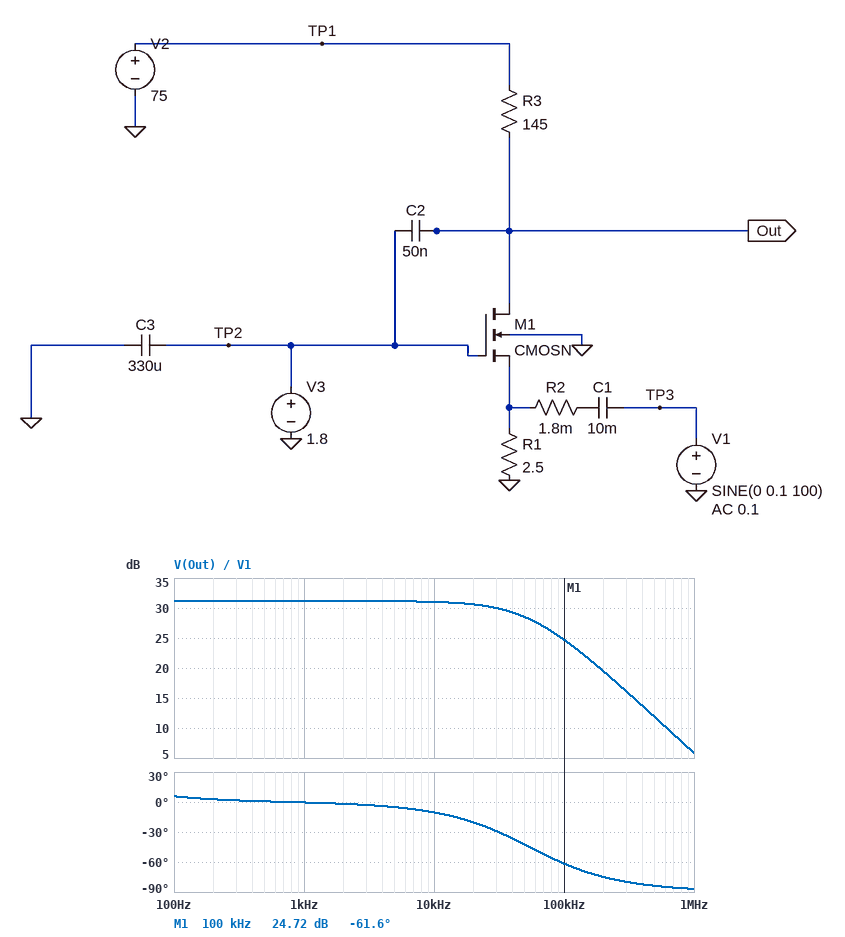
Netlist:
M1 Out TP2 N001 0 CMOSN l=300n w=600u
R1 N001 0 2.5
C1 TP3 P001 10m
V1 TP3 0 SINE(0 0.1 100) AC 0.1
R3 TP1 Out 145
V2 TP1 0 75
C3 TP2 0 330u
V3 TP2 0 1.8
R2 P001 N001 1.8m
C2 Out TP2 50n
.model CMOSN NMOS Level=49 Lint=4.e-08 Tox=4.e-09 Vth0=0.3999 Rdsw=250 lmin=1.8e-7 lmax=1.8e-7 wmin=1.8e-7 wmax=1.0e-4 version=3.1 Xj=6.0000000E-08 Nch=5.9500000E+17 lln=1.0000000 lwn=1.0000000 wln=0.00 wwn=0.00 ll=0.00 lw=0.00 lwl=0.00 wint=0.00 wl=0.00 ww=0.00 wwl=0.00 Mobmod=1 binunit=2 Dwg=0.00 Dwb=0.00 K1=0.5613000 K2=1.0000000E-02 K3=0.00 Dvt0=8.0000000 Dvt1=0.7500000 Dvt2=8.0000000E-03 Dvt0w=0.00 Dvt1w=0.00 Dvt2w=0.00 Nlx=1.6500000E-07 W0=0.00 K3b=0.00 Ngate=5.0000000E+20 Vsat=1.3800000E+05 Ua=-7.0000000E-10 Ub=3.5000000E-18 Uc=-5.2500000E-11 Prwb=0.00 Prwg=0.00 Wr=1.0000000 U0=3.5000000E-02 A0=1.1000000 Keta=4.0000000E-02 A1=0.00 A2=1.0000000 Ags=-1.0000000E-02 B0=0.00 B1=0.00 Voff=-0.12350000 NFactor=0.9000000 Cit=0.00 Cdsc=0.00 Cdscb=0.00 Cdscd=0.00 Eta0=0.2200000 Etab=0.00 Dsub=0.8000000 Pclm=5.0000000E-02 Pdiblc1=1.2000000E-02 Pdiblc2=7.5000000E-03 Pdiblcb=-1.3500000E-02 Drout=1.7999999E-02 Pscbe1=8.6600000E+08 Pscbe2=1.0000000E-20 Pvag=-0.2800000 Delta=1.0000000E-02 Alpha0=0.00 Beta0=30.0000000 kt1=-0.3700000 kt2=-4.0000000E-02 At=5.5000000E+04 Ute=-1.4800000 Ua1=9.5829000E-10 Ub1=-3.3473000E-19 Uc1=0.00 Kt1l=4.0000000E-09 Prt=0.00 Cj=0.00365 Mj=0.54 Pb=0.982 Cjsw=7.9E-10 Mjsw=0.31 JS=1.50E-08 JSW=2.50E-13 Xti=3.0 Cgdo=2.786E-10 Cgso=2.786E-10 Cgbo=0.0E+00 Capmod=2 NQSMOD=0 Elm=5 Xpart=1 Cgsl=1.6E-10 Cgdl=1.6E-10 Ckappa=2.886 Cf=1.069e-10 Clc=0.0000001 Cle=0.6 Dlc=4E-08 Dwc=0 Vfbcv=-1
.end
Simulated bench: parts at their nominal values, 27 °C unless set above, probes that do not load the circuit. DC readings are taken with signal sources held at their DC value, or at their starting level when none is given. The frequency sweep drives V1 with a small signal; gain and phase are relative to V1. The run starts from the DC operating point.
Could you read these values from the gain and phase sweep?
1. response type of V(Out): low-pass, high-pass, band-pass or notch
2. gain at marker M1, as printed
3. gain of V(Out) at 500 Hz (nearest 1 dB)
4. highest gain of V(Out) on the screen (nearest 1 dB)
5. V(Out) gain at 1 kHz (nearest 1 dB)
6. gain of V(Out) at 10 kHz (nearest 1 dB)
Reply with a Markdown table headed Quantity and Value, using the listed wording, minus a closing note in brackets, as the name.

| Quantity | Value |
|---|---|
| response type of V(Out): low-pass, high-pass, band-pass or notch | low-pass |
| gain at marker M1, as printed | 24.72 dB |
| gain of V(Out) at 500 Hz | 31 dB |
| highest gain of V(Out) on the screen | 31 dB |
| V(Out) gain at 1 kHz | 31 dB |
| gain of V(Out) at 10 kHz | 31 dB |
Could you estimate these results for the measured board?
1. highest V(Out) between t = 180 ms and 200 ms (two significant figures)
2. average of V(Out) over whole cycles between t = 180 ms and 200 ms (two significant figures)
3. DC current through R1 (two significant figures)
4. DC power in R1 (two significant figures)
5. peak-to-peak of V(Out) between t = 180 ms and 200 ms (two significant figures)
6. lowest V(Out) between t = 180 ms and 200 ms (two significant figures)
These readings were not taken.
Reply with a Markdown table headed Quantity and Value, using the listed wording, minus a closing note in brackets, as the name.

| Quantity | Value |
|---|---|
| highest V(Out) between t = 180 ms and 200 ms | 38 V |
| average of V(Out) over whole cycles between t = 180 ms and 200 ms | 34 V |
| DC current through R1 | 280 mA |
| DC power in R1 | 200 mW |
| peak-to-peak of V(Out) between t = 180 ms and 200 ms | 7.2 V |
| lowest V(Out) between t = 180 ms and 200 ms | 30 V |
